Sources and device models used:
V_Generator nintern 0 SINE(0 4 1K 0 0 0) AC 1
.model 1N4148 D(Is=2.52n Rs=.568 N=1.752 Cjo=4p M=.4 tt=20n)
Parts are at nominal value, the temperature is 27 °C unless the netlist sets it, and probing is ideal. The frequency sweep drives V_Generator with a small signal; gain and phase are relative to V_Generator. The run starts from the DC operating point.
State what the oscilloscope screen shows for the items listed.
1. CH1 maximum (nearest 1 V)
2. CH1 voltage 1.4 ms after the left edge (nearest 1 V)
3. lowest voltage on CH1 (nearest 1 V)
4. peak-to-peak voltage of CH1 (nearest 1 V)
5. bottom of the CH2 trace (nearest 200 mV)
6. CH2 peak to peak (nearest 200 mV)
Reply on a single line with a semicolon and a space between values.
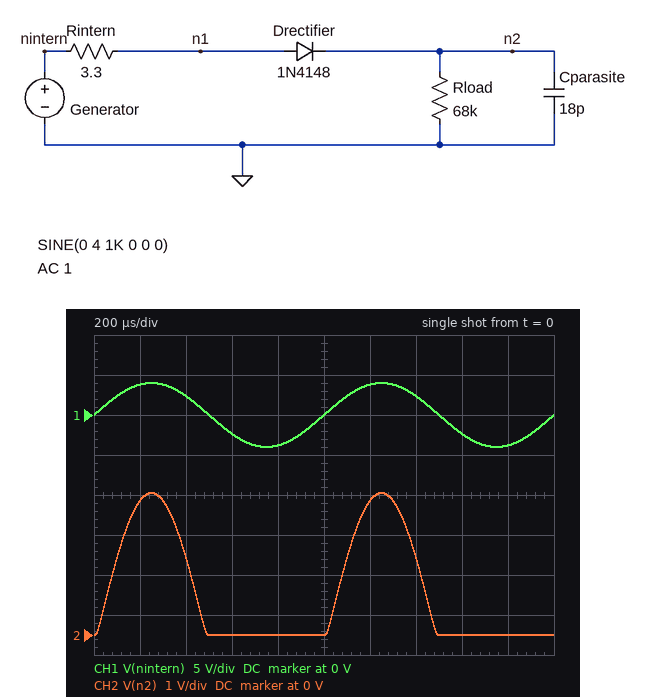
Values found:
4 V; 2 V; -4 V; 8 V; 0 V; 3.6 V
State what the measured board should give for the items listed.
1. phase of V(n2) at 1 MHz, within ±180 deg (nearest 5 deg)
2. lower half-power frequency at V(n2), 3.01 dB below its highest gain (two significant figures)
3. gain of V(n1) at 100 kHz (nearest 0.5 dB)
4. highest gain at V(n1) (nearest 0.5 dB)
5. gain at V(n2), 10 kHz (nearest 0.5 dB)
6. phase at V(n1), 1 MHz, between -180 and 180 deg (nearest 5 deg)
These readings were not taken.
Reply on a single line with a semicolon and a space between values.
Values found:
5 deg; 110 kHz; 0 dB; 0 dB; -35.0 dB; 0 deg
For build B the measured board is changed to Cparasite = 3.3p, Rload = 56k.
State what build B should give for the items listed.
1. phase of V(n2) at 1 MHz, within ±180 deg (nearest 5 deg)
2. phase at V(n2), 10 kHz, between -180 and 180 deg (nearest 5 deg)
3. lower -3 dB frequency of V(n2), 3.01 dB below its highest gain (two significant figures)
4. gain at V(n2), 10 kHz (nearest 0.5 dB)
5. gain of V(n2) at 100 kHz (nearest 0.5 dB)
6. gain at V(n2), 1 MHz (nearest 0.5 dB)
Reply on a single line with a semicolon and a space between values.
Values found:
20 deg; 75 deg; 390 kHz; -37.0 dB; -17.5 dB; -6.0 dB
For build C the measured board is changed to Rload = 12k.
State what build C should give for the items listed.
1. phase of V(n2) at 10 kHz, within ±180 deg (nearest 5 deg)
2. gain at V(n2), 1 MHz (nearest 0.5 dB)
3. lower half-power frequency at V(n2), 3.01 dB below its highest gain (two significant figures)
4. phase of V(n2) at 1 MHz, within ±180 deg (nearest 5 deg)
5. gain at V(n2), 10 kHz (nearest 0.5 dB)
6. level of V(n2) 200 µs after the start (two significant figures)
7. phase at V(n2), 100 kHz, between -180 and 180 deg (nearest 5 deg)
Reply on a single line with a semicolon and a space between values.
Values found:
75 deg; -16.0 dB; 600 kHz; 30 deg; -50.0 dB; 3.3 V; 80 deg
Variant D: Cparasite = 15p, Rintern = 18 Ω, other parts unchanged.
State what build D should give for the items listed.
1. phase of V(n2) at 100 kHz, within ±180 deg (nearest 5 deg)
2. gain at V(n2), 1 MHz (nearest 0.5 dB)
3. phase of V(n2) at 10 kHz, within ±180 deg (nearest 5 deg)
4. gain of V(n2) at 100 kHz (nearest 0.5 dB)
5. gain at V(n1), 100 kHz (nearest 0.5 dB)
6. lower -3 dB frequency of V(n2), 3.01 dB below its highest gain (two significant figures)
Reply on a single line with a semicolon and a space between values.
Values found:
50 deg; -13.5 dB; 75 deg; -17.5 dB; 0 dB; 120 kHz
